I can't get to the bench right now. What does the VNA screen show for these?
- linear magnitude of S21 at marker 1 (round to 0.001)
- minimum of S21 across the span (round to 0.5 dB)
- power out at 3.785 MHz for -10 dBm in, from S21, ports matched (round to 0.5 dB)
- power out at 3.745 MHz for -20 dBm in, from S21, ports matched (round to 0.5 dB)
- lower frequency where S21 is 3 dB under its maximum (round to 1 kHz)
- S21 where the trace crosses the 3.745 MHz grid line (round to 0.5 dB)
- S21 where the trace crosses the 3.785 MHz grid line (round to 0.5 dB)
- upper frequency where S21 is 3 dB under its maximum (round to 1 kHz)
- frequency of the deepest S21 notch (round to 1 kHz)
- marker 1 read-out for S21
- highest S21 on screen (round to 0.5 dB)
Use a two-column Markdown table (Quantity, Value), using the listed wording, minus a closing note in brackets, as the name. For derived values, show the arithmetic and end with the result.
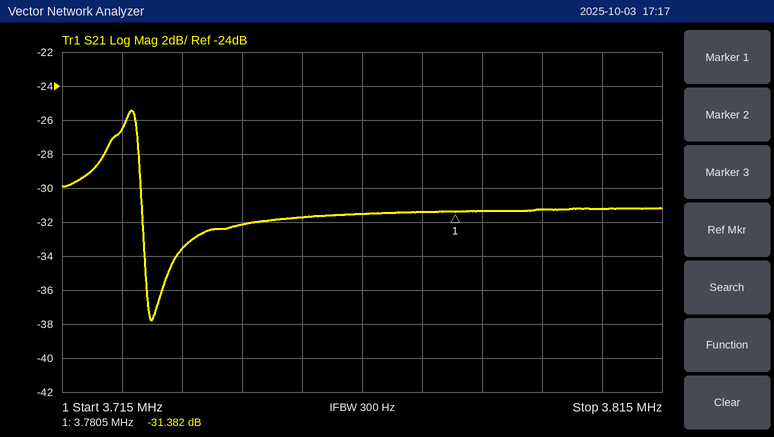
| Quantity | Value |
|---|---|
| linear magnitude of S21 at marker 1 | 10^(-31.382/20) ≈ 0.027 |
| minimum of S21 across the span | -38.0 dB |
| power out at 3.785 MHz for -10 dBm in, from S21, ports matched | -10 dBm + (-31.5 dB) = -41.5 dBm |
| power out at 3.745 MHz for -20 dBm in, from S21, ports matched | -20 dBm + (-32.0 dB) = -52.0 dBm |
| lower frequency where S21 is 3 dB under its maximum | 3.721 MHz |
| S21 where the trace crosses the 3.745 MHz grid line | -32.0 dB |
| S21 where the trace crosses the 3.785 MHz grid line | -31.5 dB |
| upper frequency where S21 is 3 dB under its maximum | 3.728 MHz |
| frequency of the deepest S21 notch | 3.730 MHz |
| marker 1 read-out for S21 | -31.382 dB |
| highest S21 on screen | -25.5 dB |
